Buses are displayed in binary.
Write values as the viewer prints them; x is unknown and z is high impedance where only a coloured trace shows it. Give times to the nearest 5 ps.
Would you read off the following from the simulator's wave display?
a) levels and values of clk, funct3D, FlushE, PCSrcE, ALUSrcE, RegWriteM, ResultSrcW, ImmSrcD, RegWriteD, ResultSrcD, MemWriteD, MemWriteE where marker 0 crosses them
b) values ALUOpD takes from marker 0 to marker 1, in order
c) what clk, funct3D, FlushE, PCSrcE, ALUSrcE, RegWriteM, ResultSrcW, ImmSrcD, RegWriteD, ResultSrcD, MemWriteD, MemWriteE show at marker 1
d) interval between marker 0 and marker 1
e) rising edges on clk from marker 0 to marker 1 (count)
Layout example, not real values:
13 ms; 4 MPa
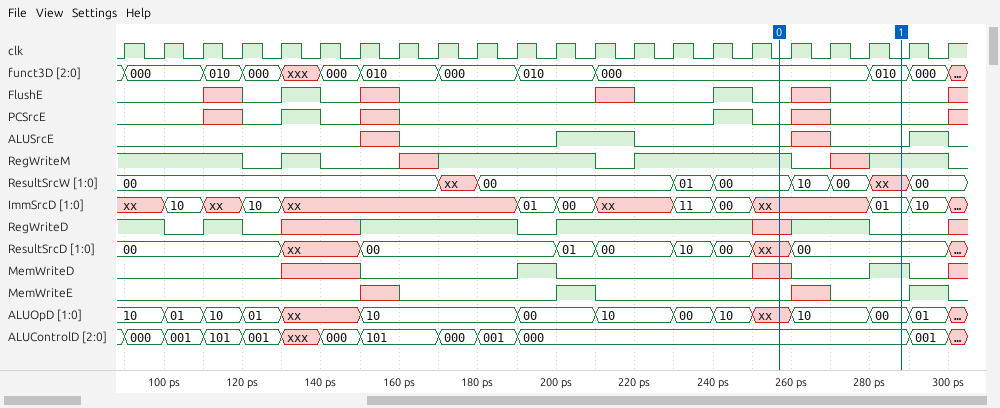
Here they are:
clk=0, funct3D=000, FlushE=0, PCSrcE=0, ALUSrcE=0, RegWriteM=1, ResultSrcW=00, ImmSrcD=xx, RegWriteD=x, ResultSrcD=xx, MemWriteD=x, MemWriteE=0; xx, 10, 00; clk=0, funct3D=010, FlushE=0, PCSrcE=0, ALUSrcE=0, RegWriteM=1, ResultSrcW=xx, ImmSrcD=01, RegWriteD=0, ResultSrcD=00, MemWriteD=1, MemWriteE=0; 30 ps; 3
